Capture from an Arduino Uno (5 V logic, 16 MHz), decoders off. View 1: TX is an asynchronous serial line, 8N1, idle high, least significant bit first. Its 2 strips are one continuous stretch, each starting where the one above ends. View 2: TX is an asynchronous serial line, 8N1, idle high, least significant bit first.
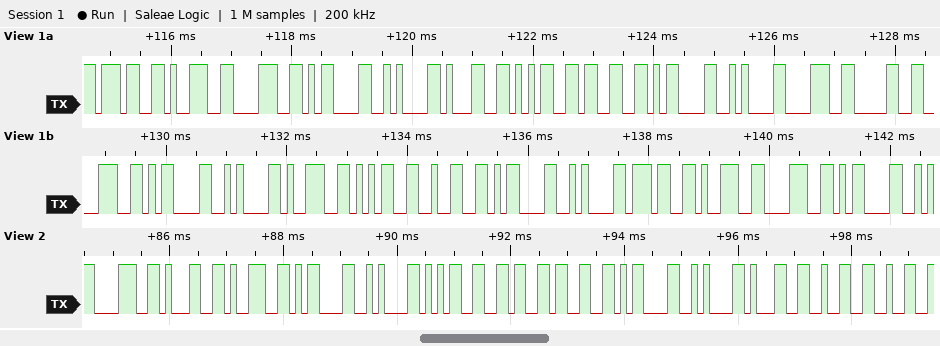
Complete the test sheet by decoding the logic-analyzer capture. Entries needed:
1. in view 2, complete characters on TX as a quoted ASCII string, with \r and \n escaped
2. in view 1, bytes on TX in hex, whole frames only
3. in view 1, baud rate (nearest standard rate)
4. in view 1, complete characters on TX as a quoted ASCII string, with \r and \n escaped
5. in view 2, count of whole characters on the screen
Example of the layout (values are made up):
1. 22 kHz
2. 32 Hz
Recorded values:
1. "819\r\n563\r\n122"
2. 37 39 38 0D 0A 31 35 33 0D 0A 38 30 38 0D 0A 39 35 32 0D 0A 37 39 38 0D
3. 9600 baud
4. "798\r\n153\r\n808\r\n952\r\n798\r"
5. 13
